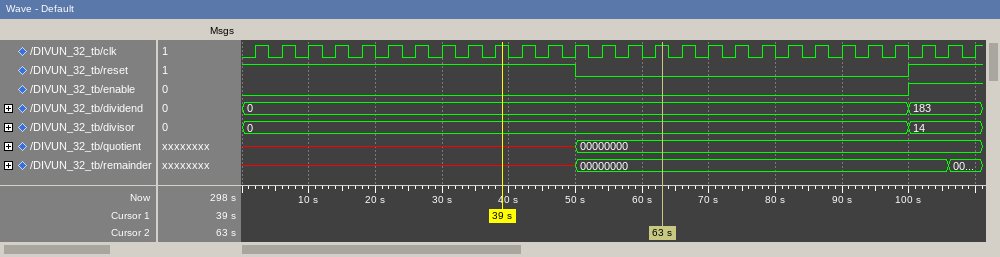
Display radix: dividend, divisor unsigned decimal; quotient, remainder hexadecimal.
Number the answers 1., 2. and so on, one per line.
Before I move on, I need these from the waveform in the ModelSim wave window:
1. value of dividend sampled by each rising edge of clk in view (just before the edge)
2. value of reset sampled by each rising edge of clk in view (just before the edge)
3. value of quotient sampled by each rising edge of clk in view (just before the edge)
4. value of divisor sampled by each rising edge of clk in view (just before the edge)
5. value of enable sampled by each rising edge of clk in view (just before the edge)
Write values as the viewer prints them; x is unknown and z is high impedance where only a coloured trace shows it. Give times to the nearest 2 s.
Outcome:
1. 0, 0, 0, 0, 0, 0, 0, 0, 0, 0, 0, 0, 0, 0, 0, 0, 0, 0, 0, 0, 0, 0, 0, 0, 0, 183, 183, 183
2. 1 1 1 1 1 1 1 1 1 1 1 1 1 0 0 0 0 0 0 0 0 0 0 0 0 1 1 1
3. x, x, x, x, x, x, x, x, x, x, x, x, x, 00000000, 00000000, 00000000, 00000000, 00000000, 00000000, 00000000, 00000000, 00000000, 00000000, 00000000, 00000000, 00000000, 00000000, 00000000
4. 0, 0, 0, 0, 0, 0, 0, 0, 0, 0, 0, 0, 0, 0, 0, 0, 0, 0, 0, 0, 0, 0, 0, 0, 0, 14, 14, 14
5. 0 0 0 0 0 0 0 0 0 0 0 0 0 0 0 0 0 0 0 0 0 0 0 0 0 1 1 1
